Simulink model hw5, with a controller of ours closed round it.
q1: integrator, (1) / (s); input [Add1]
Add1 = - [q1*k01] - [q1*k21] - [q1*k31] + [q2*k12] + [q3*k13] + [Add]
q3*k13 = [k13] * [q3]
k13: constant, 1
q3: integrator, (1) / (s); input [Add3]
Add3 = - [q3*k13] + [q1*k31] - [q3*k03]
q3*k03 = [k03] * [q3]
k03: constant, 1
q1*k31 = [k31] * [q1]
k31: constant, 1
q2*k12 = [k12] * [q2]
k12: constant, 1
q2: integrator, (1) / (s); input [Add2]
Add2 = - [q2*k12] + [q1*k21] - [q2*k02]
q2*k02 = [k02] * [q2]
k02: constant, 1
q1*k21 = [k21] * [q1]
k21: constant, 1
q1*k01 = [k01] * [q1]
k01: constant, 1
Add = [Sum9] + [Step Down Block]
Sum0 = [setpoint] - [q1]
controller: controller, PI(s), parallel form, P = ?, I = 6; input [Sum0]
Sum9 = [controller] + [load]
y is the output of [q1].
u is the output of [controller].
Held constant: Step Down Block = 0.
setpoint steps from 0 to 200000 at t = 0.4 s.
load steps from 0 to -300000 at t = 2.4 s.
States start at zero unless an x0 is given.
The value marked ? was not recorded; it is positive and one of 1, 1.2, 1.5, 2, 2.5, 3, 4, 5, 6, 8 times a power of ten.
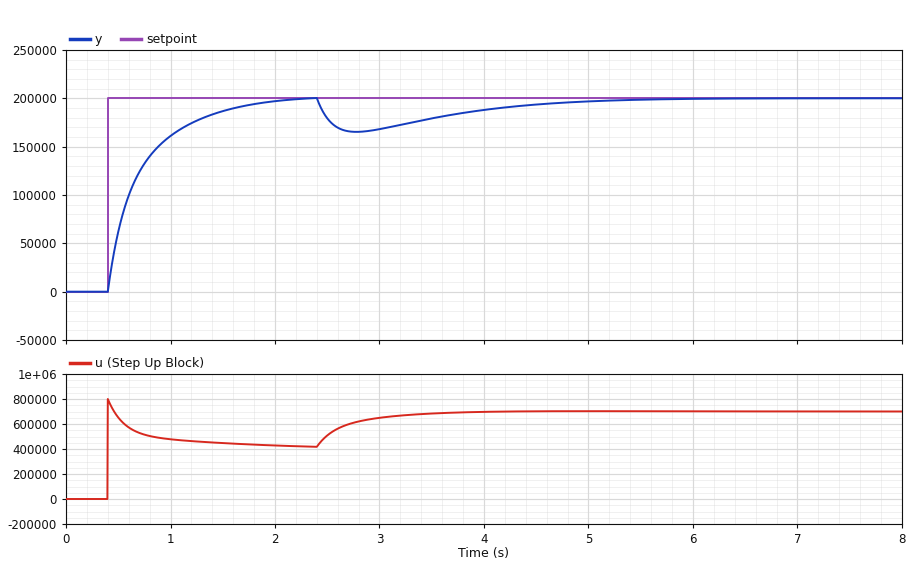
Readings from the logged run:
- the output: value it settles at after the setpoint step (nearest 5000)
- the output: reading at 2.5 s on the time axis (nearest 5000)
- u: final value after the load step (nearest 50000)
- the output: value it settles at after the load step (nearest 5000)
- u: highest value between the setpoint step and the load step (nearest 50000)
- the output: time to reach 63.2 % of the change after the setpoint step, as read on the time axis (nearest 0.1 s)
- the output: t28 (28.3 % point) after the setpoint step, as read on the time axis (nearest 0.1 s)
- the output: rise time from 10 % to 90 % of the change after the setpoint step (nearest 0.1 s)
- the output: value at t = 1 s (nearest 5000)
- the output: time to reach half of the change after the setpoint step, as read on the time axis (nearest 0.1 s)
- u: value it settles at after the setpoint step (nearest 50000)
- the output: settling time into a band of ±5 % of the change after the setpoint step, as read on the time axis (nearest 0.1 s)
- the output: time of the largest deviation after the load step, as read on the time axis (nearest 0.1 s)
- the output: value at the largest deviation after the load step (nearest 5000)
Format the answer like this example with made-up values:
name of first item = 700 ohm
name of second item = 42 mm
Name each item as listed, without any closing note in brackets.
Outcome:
the output: value it settles at after the setpoint step = 200000
the output: reading at 2.5 s on the time axis = 180000
u: final value after the load step = 700000
the output: value it settles at after the load step = 200000
u: highest value between the setpoint step and the load step = 800000
the output: time to reach 63.2 % of the change after the setpoint step, as read on the time axis = 0.7 s
the output: t28 (28.3 % point) after the setpoint step, as read on the time axis = 0.5 s
the output: rise time from 10 % to 90 % of the change after the setpoint step = 0.9 s
the output: value at t = 1 s = 160000
the output: time to reach half of the change after the setpoint step, as read on the time axis = 0.6 s
u: value it settles at after the setpoint step = 400000
the output: settling time into a band of ±5 % of the change after the setpoint step, as read on the time axis = 1.6 s
the output: time of the largest deviation after the load step, as read on the time axis = 2.8 s
the output: value at the largest deviation after the load step = 165000
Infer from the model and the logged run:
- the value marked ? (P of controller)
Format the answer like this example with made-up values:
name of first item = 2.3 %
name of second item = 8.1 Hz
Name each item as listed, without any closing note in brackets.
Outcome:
the value marked ? = 4
